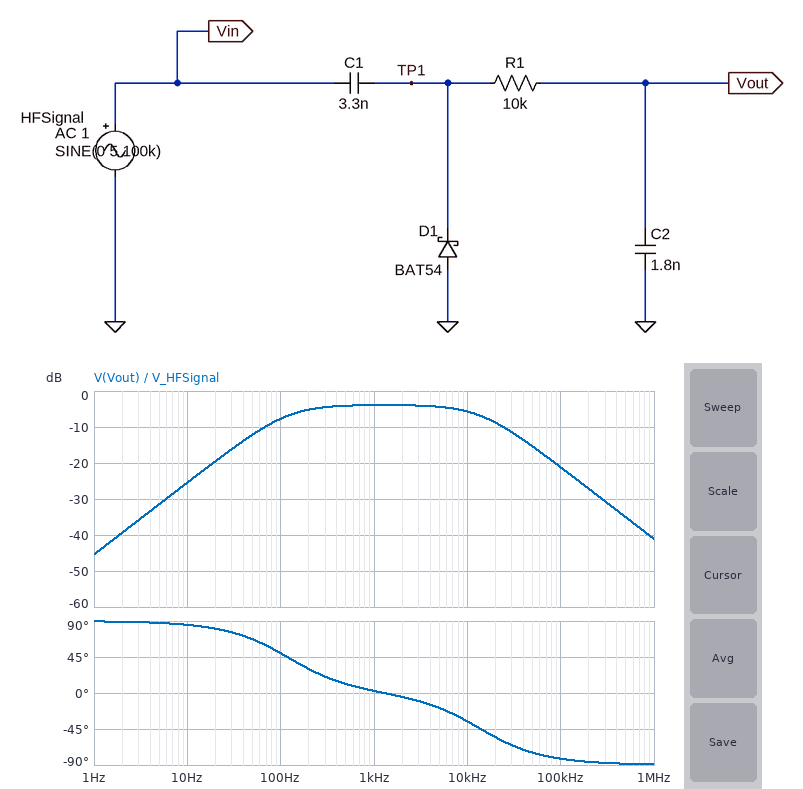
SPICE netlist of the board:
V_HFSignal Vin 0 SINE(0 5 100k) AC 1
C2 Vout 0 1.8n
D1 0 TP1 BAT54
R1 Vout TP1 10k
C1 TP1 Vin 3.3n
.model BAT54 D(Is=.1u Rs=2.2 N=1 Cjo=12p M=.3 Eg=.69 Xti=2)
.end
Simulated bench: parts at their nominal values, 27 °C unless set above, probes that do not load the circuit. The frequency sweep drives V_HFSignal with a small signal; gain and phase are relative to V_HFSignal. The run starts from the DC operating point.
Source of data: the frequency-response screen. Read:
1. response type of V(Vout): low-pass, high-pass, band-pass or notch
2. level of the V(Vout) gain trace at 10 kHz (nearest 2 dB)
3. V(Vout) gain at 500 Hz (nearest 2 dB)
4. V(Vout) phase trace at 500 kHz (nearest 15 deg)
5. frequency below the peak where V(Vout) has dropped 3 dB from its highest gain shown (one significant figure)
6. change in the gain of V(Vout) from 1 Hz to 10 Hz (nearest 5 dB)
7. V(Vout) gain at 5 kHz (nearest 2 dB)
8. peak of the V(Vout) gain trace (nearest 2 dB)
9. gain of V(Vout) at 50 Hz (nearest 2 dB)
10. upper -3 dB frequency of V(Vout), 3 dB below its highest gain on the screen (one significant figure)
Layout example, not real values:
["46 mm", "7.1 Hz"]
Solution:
["band-pass", "-6 dB", "-4 dB", "-90 deg", "100 Hz", "20 dB", "-4 dB", "-4 dB", "-12 dB", "10 kHz"]
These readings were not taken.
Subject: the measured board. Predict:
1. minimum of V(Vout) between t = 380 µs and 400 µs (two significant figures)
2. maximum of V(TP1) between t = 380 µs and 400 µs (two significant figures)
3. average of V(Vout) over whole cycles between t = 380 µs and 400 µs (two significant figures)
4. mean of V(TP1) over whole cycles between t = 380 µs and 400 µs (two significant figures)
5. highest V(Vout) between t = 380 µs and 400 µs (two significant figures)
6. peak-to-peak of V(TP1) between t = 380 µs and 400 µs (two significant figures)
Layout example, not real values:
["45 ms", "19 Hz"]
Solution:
["4.4 V", "9.8 V", "4.8 V", "4.8 V", "5.3 V", "9.9 V"]
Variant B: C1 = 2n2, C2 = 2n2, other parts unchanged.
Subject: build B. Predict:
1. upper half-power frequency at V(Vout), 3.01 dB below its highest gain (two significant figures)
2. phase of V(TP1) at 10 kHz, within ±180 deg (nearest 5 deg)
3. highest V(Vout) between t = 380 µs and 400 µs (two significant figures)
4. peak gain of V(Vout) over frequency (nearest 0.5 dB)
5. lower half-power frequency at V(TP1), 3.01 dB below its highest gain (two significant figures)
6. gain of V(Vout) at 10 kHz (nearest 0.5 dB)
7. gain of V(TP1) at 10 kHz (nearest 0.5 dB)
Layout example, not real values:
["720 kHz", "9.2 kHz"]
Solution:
["15 kHz", "20 deg", "5.2 V", "-6.0 dB", "10 kHz", "-8.0 dB", "-3.0 dB"]
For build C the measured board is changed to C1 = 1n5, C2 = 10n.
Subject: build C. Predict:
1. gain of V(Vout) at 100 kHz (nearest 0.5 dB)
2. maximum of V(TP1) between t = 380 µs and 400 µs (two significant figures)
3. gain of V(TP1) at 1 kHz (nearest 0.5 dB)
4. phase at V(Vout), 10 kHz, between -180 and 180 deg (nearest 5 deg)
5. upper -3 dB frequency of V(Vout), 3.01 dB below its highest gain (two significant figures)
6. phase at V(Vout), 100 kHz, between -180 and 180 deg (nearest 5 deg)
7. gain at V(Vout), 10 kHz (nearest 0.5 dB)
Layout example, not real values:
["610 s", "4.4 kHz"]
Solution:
["-36.0 dB", "9.6 V", "-16.5 dB", "-40 deg", "13 kHz", "-85 deg", "-20.0 dB"]
